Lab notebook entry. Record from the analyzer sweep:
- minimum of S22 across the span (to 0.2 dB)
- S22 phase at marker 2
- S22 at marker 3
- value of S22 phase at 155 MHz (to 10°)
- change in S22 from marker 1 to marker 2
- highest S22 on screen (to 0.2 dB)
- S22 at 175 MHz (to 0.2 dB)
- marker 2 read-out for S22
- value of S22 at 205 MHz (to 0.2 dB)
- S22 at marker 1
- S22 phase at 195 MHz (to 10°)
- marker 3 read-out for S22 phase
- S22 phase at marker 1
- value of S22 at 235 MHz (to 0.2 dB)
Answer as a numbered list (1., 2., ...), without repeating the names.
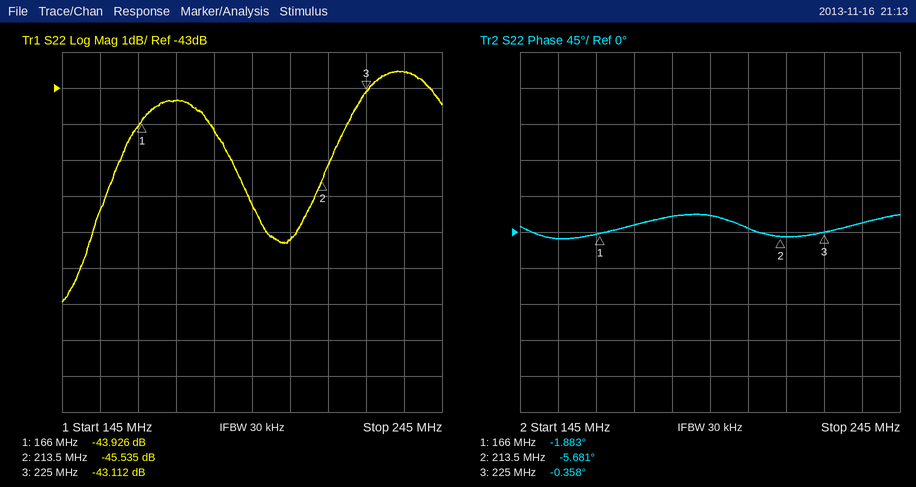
1. -49.0 dB
2. -5.681°
3. -43.112 dB
4. -10°
5. -1.609 dB
6. -42.6 dB
7. -43.4 dB
8. -45.535 dB
9. -47.2 dB
10. -43.926 dB
11. 20°
12. -0.358°
13. -1.883°
14. -42.6 dB
